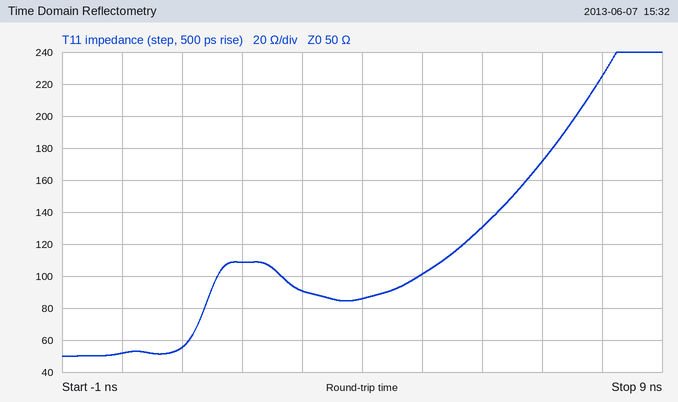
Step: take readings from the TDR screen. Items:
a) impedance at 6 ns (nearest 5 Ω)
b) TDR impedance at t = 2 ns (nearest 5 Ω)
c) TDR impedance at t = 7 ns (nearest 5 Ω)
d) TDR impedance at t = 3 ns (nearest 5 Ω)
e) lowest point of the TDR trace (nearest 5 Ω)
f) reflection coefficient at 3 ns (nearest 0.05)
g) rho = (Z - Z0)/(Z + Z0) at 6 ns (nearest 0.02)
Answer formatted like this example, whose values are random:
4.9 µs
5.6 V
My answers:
130 Ω
110 Ω
170 Ω
90 Ω
50 Ω
+0.30
+0.44
